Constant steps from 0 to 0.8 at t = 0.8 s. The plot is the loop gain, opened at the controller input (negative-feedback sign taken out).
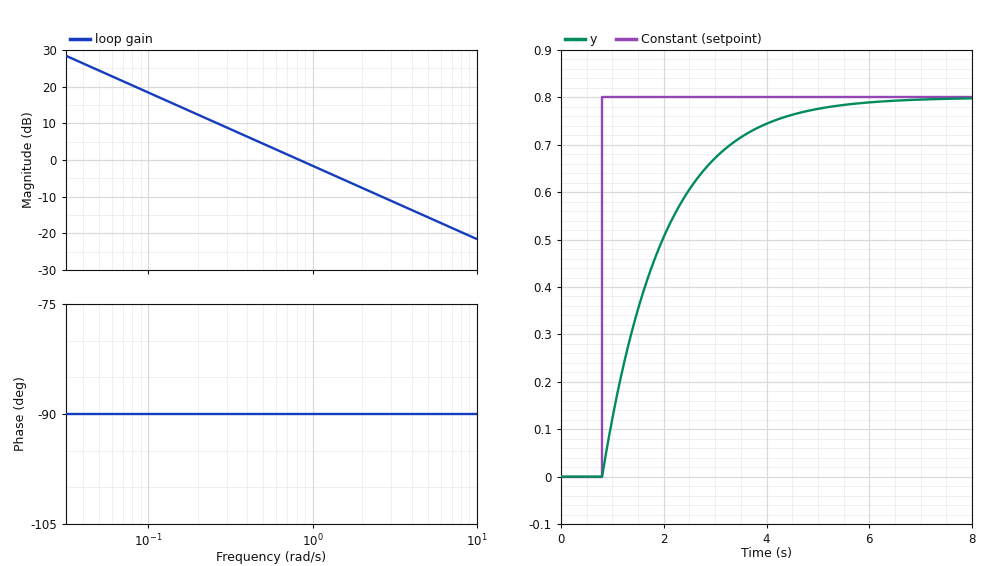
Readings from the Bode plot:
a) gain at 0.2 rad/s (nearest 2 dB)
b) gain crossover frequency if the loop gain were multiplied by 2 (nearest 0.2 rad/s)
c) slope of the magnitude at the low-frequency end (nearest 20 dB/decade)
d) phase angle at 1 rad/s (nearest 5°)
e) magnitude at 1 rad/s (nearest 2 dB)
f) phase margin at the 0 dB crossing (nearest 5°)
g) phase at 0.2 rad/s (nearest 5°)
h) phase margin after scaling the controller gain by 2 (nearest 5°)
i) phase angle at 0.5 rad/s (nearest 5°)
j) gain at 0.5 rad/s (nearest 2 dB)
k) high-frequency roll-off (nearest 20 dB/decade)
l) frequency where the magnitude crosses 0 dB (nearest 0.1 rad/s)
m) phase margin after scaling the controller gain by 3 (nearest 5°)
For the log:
12 dB
1.6 rad/s
-20 dB/decade
-90°
-2 dB
90°
-90°
90°
-90°
4 dB
-20 dB/decade
0.8 rad/s
90°
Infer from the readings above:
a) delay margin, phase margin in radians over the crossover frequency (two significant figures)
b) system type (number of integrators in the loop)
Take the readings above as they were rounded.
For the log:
2.0 s
1
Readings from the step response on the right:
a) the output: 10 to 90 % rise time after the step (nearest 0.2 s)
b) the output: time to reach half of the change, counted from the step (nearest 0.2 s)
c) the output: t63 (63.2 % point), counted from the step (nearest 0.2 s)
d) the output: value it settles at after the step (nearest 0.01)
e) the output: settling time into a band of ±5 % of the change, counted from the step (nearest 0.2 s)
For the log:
2.6 s
0.8 s
1.2 s
0.80
3.6 s
